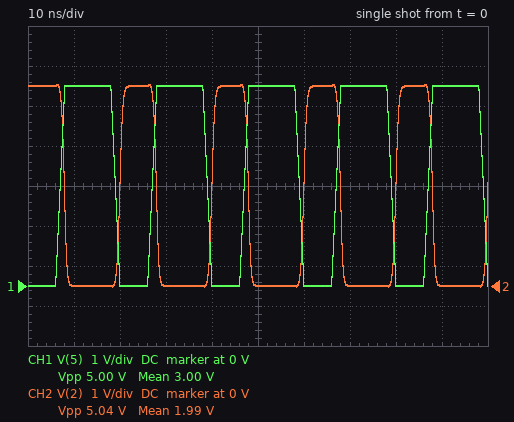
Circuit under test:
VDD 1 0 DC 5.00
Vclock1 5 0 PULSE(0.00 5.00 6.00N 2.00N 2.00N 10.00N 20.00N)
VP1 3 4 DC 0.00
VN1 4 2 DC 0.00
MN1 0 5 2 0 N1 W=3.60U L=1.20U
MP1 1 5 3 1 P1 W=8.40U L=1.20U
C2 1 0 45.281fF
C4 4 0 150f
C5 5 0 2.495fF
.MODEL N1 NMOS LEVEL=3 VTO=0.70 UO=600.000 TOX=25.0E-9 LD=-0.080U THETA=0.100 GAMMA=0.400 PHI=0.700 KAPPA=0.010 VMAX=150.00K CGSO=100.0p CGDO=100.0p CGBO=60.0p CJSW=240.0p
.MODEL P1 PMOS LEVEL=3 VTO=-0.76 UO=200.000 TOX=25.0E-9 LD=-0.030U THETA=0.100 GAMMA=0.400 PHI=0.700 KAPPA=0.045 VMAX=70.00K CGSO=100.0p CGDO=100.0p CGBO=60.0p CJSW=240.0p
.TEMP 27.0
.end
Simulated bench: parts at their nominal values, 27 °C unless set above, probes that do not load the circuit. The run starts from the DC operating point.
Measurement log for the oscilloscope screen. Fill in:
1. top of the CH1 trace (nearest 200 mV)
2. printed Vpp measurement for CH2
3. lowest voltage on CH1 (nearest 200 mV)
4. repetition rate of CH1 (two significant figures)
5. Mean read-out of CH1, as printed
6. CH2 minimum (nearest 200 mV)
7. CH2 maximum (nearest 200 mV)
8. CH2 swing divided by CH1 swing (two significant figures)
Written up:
5.0 V
5.04 V
0 V
50 MHz
3.00 V
0 V
5.0 V
1.0
